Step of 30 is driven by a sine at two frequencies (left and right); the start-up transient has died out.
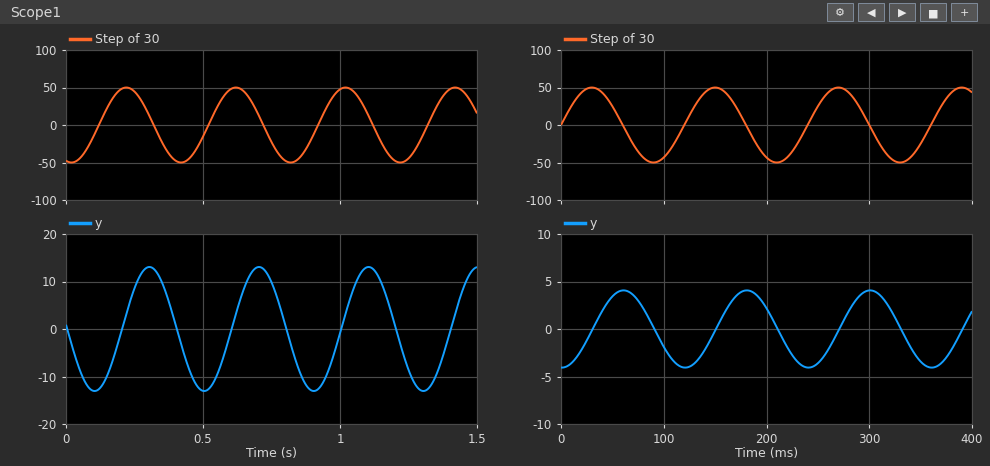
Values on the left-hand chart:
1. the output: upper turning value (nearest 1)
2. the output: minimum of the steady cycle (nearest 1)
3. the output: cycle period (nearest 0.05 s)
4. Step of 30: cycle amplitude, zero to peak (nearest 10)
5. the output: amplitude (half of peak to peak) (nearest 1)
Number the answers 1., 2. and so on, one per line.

1. 13
2. -13
3. 0.40 s
4. 50
5. 13
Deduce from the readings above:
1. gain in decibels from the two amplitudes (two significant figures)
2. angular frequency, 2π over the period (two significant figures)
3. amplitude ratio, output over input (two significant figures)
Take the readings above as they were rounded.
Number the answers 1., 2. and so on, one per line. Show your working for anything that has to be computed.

1. 20 log10(13 / 50) = -12 dB
2. 2π / 0.4 = 16 rad/s
3. 13 / 50 = 0.26
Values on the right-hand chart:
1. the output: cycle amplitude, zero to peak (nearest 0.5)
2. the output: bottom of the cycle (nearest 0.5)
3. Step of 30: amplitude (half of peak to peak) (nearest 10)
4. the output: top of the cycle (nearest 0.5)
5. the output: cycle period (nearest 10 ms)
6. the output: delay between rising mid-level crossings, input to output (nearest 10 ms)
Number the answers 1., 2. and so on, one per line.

1. 4.0
2. -4.0
3. 50
4. 4.0
5. 120 ms
6. 30 ms
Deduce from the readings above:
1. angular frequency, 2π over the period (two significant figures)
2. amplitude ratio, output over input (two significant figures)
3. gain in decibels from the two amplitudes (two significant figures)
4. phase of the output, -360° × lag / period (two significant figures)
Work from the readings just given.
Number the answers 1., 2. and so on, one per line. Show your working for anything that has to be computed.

1. 2π / 120 = 0.052 rad/ms
2. 4 / 50 = 0.080
3. 20 log10(4 / 50) = -22 dB
4. -360 × 30 / 120 = -90°
